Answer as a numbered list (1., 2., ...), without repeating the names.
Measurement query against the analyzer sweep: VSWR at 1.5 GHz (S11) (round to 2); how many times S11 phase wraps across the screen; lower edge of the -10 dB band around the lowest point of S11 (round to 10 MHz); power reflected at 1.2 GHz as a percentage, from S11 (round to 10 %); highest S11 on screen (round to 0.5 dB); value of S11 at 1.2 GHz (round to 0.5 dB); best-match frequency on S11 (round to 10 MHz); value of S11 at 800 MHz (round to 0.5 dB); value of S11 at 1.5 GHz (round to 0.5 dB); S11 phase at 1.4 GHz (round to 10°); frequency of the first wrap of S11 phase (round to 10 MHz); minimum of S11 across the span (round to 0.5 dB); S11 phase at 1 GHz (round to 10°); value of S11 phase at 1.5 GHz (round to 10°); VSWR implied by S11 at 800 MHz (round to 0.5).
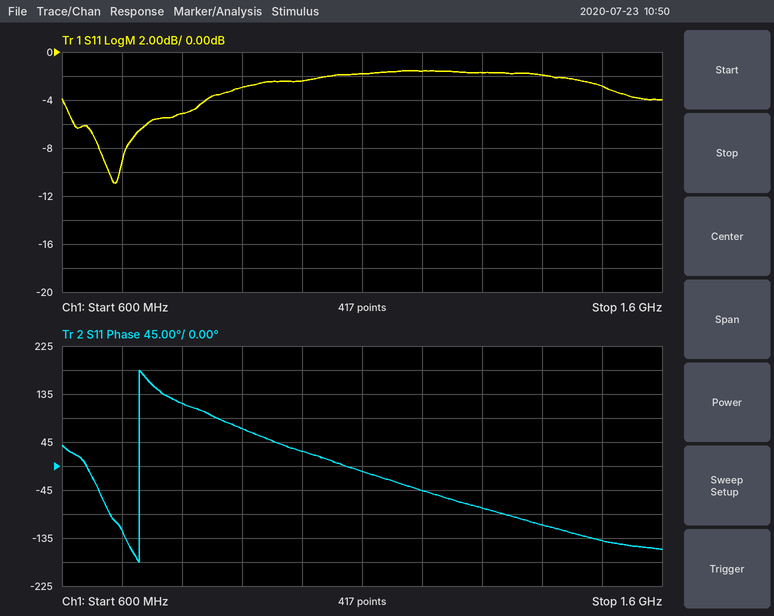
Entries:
1. 6
2. 1
3. 680 MHz
4. 70 %
5. -1.5 dB
6. -1.5 dB
7. 690 MHz
8. -5.0 dB
9. -3.0 dB
10. -110°
11. 730 MHz
12. -11.0 dB
13. 30°
14. -140°
15. 3.5
